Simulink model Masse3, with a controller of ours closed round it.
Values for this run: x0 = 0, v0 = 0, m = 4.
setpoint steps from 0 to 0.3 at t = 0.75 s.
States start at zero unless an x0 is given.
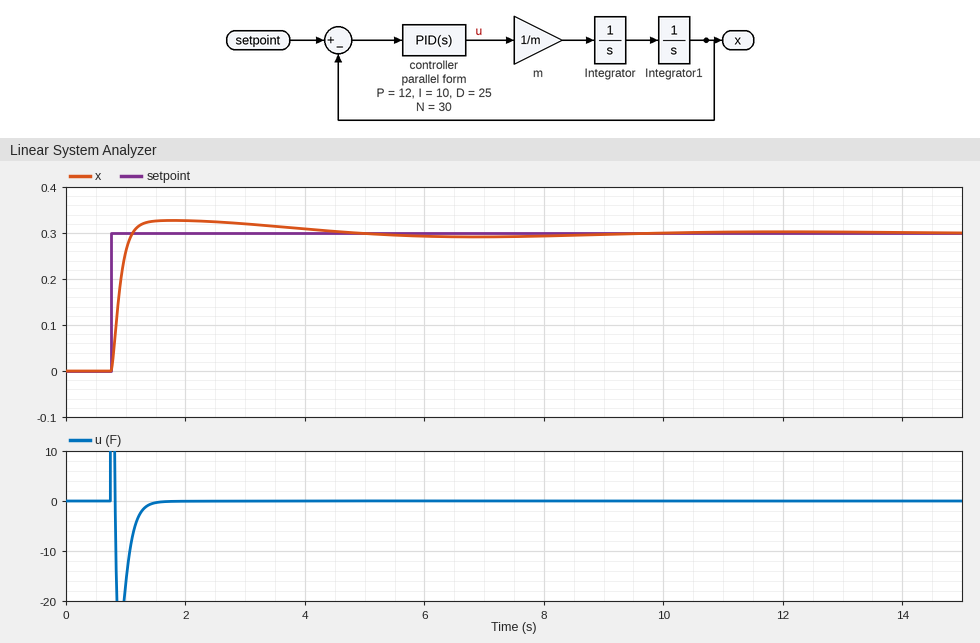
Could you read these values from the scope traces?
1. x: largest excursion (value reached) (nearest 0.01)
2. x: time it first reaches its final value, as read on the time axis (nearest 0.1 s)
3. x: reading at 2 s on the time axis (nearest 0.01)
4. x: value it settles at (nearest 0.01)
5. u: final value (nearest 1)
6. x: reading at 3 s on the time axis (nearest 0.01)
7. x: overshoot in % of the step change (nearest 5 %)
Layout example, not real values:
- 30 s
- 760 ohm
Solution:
- 0.33
- 1.1 s
- 0.33
- 0.30
- 0
- 0.32
- 10 %
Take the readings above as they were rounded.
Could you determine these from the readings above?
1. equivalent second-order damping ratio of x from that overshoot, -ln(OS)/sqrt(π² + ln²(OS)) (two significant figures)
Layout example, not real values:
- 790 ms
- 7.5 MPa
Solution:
- 0.59
